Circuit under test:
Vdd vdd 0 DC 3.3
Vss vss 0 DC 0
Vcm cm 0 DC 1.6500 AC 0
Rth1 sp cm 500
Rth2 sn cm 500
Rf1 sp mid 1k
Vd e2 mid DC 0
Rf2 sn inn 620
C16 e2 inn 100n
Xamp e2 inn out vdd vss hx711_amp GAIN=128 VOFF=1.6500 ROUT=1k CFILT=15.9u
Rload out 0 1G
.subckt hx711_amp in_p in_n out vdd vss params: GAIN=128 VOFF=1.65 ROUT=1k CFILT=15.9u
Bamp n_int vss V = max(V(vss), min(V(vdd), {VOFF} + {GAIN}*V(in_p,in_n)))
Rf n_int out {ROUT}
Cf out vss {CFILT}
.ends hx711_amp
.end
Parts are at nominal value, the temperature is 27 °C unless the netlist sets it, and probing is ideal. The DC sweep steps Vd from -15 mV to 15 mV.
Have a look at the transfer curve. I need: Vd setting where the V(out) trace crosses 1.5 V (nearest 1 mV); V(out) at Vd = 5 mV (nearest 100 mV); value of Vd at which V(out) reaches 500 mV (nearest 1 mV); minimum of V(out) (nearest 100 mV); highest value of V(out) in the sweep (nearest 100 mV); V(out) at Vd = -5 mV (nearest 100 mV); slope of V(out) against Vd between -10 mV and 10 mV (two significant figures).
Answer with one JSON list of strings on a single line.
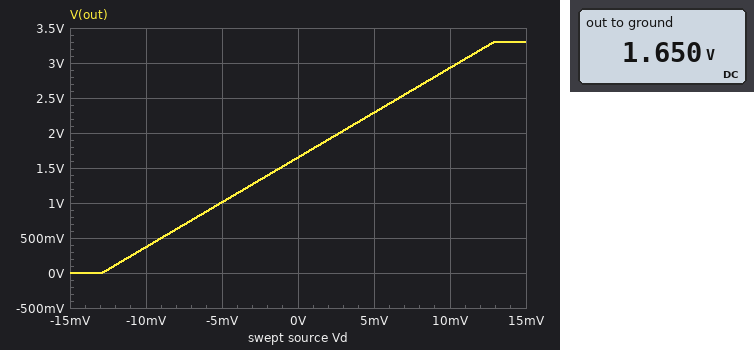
["-1 mV", "2.3 V", "-9 mV", "0 V", "3.3 V", "1.0 V", "130 V/V"]
